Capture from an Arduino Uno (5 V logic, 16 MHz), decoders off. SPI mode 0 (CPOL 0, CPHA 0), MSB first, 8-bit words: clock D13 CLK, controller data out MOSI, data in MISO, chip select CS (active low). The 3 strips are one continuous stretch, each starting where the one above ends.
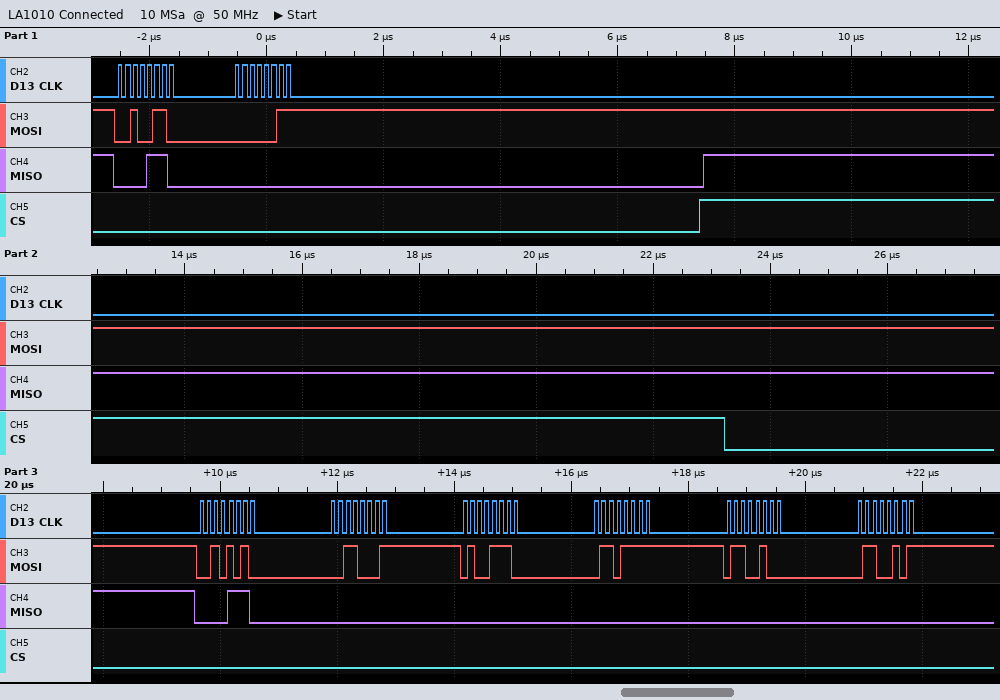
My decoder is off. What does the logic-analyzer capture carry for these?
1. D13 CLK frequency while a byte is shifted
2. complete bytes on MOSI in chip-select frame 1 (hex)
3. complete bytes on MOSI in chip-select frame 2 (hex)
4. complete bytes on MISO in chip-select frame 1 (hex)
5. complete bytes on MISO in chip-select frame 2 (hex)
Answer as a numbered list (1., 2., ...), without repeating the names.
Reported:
1. 8 MHz
2. 0x26 0x03
3. 0x2A 0x31 0x4E 0x6F 0x64 0x65
4. 0x0E 0x00
5. 0x0E 0x00 0x00 0x00 0x00 0x00
